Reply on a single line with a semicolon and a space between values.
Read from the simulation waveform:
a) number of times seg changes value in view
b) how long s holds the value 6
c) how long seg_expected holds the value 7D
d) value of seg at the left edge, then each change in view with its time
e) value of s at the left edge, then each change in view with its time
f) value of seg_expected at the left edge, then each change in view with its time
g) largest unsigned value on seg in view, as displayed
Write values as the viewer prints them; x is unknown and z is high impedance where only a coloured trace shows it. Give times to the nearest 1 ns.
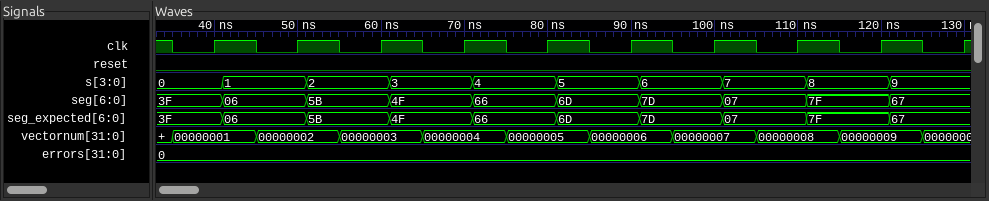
9; 10 ns; 10 ns; 3F, 06 at 41 ns, 5B at 51 ns, 4F at 61 ns, 66 at 71 ns, 6D at 81 ns, 7D at 91 ns, 07 at 101 ns, 7F at 111 ns, 67 at 121 ns; 0, 1 at 41 ns, 2 at 51 ns, 3 at 61 ns, 4 at 71 ns, 5 at 81 ns, 6 at 91 ns, 7 at 101 ns, 8 at 111 ns, 9 at 121 ns; 3F, 06 at 41 ns, 5B at 51 ns, 4F at 61 ns, 66 at 71 ns, 6D at 81 ns, 7D at 91 ns, 07 at 101 ns, 7F at 111 ns, 67 at 121 ns; 7F
